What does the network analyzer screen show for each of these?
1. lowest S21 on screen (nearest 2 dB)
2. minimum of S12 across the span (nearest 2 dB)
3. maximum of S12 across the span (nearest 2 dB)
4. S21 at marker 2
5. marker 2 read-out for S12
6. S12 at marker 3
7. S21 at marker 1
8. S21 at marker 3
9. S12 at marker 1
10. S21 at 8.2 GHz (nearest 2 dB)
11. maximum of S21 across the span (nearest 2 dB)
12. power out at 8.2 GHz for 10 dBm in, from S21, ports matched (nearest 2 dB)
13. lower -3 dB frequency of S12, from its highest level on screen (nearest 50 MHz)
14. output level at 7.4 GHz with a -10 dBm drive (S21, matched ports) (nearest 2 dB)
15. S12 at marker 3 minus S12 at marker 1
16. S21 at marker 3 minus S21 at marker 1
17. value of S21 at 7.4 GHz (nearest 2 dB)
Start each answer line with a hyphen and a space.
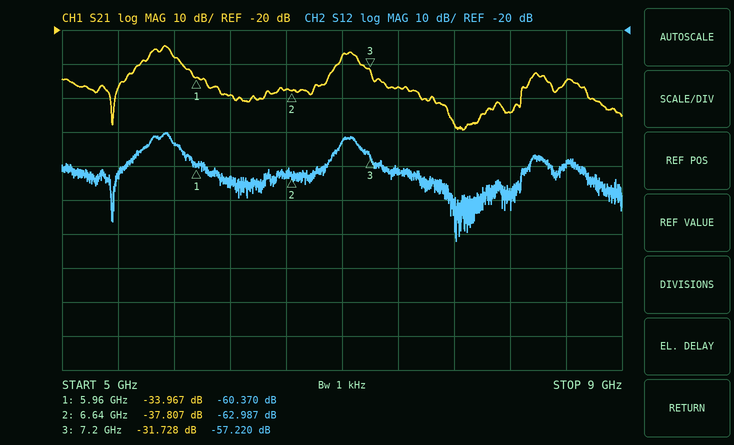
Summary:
- -50 dB
- -82 dB
- -50 dB
- -37.807 dB
- -62.987 dB
- -57.220 dB
- -33.967 dB
- -31.728 dB
- -60.370 dB
- -44 dB
- -24 dB
- -34 dBm
- 5.65 GHz
- -46 dBm
- 3.150 dB
- 2.239 dB
- -36 dB
